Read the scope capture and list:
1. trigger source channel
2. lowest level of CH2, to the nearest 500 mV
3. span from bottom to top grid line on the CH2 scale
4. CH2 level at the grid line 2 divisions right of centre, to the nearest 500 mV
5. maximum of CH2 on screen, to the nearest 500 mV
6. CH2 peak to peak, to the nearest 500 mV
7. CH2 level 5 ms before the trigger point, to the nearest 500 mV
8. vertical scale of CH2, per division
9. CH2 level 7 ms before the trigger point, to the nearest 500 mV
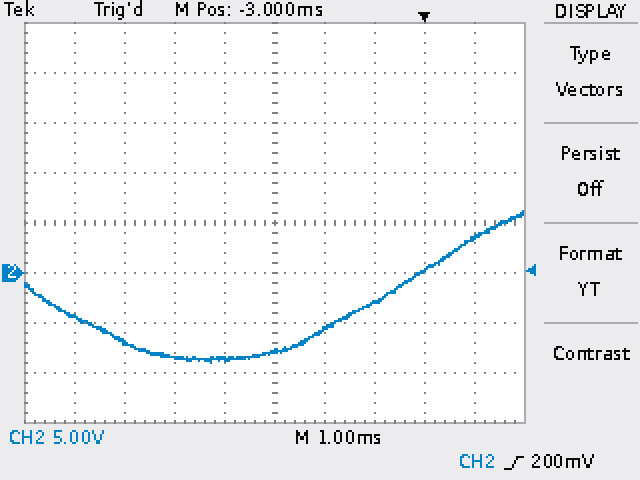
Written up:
CH2
-9.0 V
40 V
-3.0 V
6.0 V
15.0 V
-8.5 V
5 V
-4.5 V
